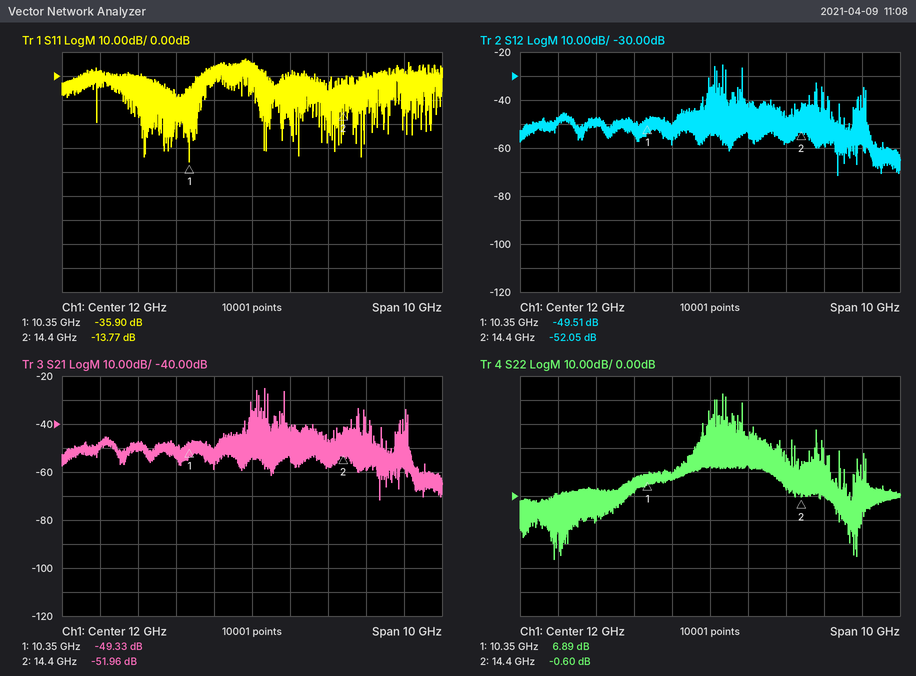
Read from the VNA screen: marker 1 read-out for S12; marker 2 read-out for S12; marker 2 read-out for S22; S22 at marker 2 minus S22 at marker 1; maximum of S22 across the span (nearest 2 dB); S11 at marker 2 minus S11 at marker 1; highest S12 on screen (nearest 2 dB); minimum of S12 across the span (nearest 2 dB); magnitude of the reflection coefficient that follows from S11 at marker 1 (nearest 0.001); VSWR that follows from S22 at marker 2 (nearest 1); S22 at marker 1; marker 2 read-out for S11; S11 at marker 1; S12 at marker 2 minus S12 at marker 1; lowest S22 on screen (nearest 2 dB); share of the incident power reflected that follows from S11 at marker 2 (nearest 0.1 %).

-49.51 dB
-52.05 dB
-0.60 dB
-7.49 dB
42 dB
22.13 dB
-26 dB
-72 dB
0.016
29
6.89 dB
-13.77 dB
-35.90 dB
-2.54 dB
-26 dB
4.2 %
